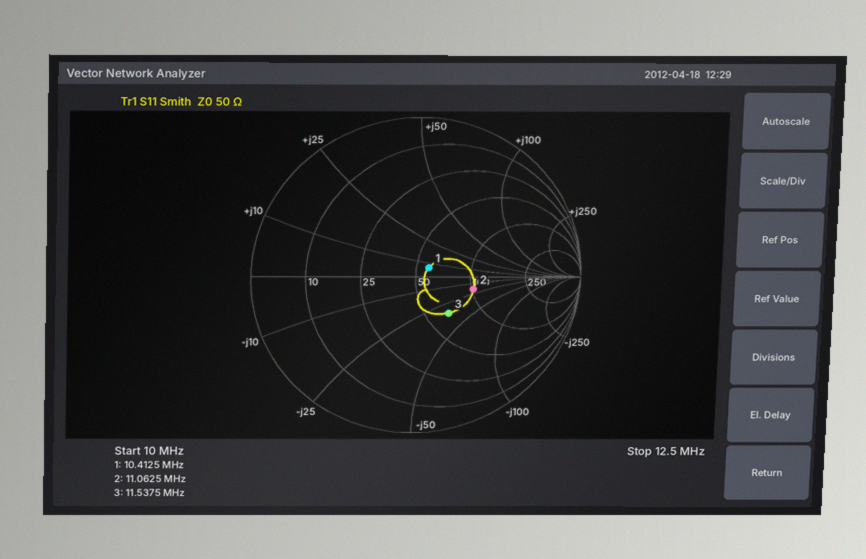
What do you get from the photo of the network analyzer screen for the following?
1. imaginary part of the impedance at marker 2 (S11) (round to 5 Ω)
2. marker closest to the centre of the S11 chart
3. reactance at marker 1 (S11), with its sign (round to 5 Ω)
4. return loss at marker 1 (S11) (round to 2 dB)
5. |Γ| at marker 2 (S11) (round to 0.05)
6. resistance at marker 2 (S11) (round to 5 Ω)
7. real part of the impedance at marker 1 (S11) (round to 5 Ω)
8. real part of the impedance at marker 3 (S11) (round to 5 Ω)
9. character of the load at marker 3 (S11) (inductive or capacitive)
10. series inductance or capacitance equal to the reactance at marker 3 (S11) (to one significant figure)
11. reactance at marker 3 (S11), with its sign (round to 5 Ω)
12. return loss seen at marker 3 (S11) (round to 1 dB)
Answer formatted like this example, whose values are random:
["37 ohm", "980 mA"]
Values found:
["-20 Ω", "marker 1", "+5 Ω", "20 dB", "0.35", "100 Ω", "60 Ω", "65 Ω", "capacitive", "400 pF", "-35 Ω", "10 dB"]
